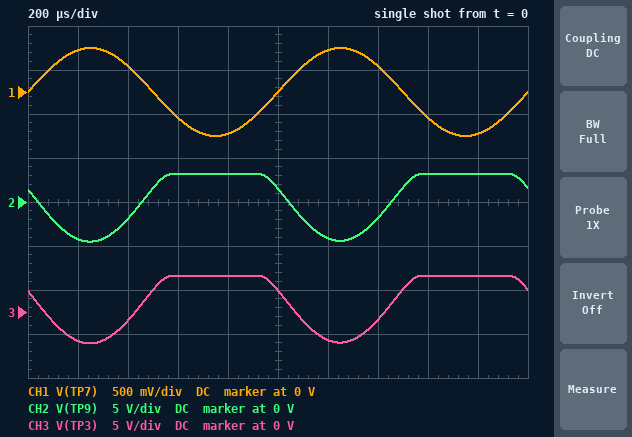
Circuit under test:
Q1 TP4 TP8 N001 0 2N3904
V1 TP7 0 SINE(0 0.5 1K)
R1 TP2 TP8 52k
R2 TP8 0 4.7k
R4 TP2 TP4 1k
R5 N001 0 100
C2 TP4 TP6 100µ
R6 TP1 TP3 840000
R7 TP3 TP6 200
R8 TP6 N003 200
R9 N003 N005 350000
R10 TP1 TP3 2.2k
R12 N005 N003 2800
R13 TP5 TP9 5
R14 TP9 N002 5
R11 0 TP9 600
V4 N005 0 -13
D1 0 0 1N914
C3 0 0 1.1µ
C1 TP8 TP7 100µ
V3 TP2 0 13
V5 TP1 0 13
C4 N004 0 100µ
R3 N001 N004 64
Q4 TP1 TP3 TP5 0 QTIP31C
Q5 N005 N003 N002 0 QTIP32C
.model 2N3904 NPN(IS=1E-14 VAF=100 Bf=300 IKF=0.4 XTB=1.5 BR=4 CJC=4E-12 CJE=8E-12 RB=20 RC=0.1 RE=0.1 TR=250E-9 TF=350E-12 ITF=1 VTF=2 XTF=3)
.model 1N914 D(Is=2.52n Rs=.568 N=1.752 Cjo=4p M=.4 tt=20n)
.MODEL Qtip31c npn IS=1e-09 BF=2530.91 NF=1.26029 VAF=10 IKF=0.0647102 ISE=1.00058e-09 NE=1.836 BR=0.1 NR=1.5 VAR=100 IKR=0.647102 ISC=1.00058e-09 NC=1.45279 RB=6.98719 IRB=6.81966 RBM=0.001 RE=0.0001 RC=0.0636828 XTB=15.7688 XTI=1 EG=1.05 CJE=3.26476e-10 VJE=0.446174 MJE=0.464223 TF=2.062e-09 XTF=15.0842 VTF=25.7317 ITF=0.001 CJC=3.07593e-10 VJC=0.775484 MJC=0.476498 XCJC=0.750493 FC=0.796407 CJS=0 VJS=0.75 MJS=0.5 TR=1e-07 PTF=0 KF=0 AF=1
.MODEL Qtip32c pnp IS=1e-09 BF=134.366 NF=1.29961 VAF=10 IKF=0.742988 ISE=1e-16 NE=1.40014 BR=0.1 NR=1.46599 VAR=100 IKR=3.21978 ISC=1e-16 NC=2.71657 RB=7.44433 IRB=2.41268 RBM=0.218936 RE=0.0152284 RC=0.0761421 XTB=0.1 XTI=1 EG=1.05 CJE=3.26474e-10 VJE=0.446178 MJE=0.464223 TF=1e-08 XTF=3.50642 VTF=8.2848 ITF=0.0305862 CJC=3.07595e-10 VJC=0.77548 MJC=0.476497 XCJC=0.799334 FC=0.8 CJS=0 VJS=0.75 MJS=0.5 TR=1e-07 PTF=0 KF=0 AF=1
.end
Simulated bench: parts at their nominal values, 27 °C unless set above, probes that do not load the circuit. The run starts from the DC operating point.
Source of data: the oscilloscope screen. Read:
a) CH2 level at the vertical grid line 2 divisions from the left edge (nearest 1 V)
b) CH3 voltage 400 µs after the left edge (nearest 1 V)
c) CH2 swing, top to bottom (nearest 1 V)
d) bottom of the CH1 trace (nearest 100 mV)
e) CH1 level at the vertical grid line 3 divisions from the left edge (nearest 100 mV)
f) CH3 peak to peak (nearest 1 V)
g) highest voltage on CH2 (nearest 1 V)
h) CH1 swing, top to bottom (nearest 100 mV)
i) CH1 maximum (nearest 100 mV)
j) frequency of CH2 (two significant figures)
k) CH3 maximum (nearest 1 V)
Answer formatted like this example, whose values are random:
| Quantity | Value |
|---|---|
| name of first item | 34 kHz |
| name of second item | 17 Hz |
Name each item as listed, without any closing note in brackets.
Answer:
| Quantity | Value |
|---|---|
| CH2 level at the vertical grid line 2 divisions from the left edge | -2 V |
| CH3 voltage 400 µs after the left edge | -1 V |
| CH2 swing, top to bottom | 8 V |
| bottom of the CH1 trace | -500 mV |
| CH1 level at the vertical grid line 3 divisions from the left edge | -300 mV |
| CH3 peak to peak | 8 V |
| highest voltage on CH2 | 3 V |
| CH1 swing, top to bottom | 1.0 V |
| CH1 maximum | 500 mV |
| frequency of CH2 | 1.0 kHz |
| CH3 maximum | 4 V |
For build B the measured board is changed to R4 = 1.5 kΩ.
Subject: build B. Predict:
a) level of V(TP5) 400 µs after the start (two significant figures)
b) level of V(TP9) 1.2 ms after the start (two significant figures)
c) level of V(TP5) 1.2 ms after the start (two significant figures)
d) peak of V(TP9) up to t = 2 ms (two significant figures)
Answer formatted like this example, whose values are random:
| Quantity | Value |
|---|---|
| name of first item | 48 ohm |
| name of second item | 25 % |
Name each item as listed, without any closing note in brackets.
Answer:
| Quantity | Value |
|---|---|
| level of V(TP5) 400 µs after the start | -2.3 V |
| level of V(TP9) 1.2 ms after the start | -5.0 V |
| level of V(TP5) 1.2 ms after the start | -4.6 V |
| peak of V(TP9) up to t = 2 ms | 3.6 V |
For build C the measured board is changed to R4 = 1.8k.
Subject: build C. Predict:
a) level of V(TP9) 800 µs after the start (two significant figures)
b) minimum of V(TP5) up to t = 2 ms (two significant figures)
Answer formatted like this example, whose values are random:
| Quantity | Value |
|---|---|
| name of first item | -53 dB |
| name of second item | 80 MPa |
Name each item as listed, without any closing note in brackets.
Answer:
| Quantity | Value |
|---|---|
| level of V(TP9) 800 µs after the start | 3.8 V |
| minimum of V(TP5) up to t = 2 ms | -3.8 V |
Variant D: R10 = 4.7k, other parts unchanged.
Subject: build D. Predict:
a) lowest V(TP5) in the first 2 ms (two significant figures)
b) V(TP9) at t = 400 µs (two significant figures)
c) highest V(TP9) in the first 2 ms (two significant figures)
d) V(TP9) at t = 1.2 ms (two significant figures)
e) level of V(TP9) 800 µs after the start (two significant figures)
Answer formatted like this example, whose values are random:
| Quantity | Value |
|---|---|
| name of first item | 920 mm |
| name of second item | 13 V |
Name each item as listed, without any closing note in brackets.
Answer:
| Quantity | Value |
|---|---|
| lowest V(TP5) in the first 2 ms | -10 V |
| V(TP9) at t = 400 µs | -6.9 V |
| highest V(TP9) in the first 2 ms | -950 mV |
| V(TP9) at t = 1.2 ms | -9.6 V |
| level of V(TP9) 800 µs after the start | -960 mV |
